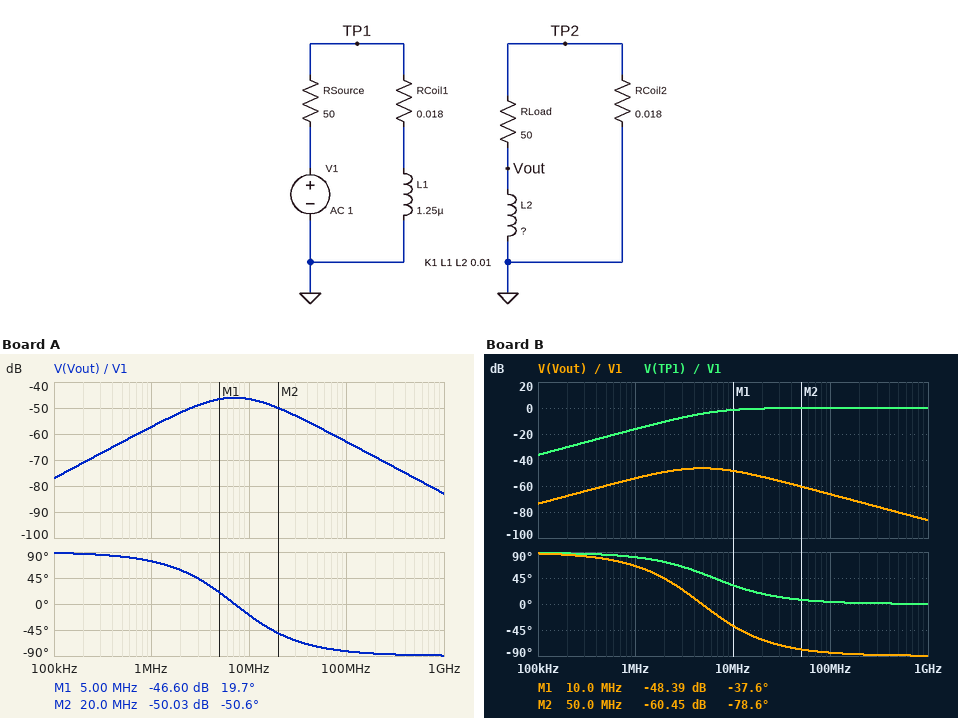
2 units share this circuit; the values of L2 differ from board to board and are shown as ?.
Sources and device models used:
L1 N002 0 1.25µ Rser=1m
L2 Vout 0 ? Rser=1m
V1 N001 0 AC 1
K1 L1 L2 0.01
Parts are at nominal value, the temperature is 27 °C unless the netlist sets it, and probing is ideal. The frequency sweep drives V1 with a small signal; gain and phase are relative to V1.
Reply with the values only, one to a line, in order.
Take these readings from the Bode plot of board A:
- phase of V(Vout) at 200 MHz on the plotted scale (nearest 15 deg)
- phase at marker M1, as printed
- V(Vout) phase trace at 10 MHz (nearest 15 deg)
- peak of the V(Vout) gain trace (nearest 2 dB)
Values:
-90 deg
19.7 deg
-15 deg
-46 dB
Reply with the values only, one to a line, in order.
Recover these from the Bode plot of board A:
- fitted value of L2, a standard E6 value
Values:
1 µH
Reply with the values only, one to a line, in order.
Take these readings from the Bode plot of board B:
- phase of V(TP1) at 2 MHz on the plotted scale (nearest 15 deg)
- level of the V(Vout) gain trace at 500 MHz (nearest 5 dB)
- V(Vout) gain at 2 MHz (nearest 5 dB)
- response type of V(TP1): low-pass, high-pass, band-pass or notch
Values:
75 deg
-80 dB
-50 dB
high-pass
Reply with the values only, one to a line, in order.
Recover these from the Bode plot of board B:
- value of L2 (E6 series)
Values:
2.2 µH
